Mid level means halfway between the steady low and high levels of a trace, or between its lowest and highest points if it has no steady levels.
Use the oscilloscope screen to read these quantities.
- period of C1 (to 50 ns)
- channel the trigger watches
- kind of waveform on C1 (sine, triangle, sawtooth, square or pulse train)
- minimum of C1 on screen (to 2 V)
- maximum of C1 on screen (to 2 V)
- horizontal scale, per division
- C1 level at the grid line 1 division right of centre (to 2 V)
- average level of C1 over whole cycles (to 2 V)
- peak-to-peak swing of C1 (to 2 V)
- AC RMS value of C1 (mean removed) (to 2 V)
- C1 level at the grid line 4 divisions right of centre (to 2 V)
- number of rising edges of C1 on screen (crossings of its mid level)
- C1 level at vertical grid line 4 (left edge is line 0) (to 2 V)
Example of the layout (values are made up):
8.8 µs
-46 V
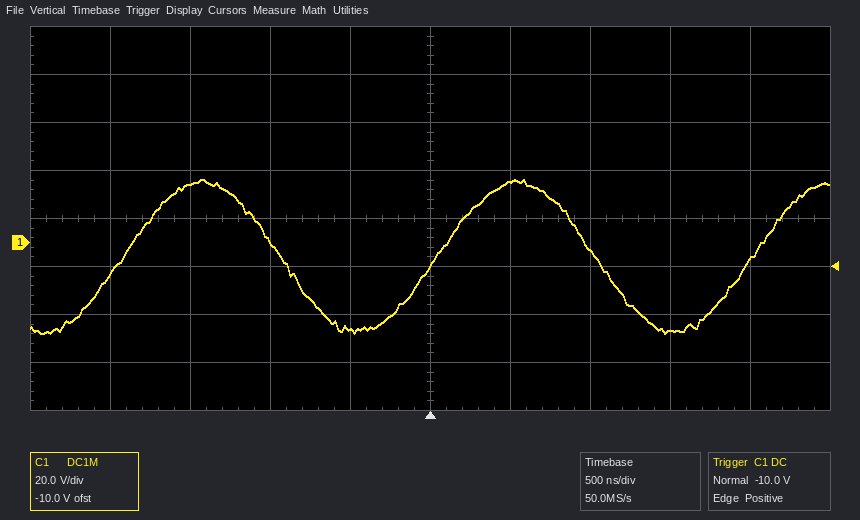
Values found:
1.95 µs
C1
sine
-38 V
26 V
500 ns
26 V
-6 V
64 V
22 V
-8 V
3
-36 V
